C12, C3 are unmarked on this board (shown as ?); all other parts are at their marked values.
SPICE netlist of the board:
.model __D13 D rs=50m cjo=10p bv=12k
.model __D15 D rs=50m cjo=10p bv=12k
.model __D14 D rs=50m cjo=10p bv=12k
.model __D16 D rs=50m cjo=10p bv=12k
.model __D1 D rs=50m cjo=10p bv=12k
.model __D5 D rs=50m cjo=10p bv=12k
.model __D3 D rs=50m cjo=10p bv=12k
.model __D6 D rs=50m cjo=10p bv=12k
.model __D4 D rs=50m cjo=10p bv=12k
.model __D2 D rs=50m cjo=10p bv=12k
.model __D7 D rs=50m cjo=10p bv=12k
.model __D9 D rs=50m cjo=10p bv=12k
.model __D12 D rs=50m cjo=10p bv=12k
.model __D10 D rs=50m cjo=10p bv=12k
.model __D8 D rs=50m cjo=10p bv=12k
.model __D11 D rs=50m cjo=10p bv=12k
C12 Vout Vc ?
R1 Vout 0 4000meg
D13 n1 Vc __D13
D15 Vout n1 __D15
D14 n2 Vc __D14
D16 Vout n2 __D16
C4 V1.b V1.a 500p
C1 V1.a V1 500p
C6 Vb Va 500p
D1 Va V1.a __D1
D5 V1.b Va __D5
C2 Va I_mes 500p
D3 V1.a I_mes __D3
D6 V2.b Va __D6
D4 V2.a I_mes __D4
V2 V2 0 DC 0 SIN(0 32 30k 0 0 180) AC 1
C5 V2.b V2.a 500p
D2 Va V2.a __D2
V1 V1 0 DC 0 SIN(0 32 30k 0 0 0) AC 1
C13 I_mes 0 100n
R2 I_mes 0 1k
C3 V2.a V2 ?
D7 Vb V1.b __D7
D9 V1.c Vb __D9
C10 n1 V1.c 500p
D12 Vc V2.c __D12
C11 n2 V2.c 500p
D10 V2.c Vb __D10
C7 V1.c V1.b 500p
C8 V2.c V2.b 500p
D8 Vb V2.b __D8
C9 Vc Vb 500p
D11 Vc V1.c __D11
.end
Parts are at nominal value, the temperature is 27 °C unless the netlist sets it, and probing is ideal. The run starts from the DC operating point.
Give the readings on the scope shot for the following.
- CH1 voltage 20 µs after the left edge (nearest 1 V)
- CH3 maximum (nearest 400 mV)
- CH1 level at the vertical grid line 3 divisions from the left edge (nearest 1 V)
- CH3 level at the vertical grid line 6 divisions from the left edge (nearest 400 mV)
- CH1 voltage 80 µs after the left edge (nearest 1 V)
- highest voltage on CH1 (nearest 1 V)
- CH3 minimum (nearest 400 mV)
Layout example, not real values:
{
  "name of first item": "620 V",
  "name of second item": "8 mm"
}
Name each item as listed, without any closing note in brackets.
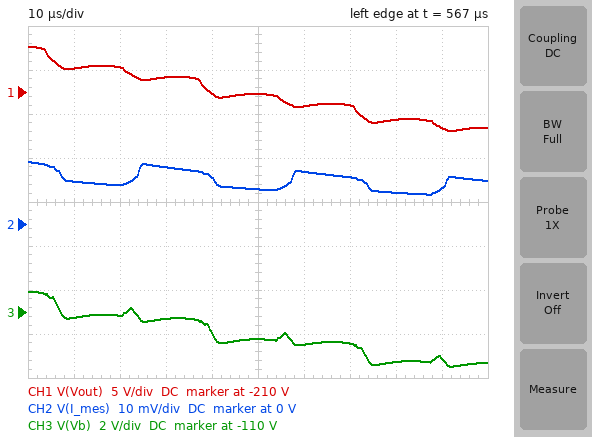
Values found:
{
  "CH1 voltage 20 µs after the left edge": "-207 V",
  "CH3 maximum": "-109.2 V",
  "CH1 level at the vertical grid line 3 divisions from the left edge": "-208 V",
  "CH3 level at the vertical grid line 6 divisions from the left edge": "-111.6 V",
  "CH1 voltage 80 µs after the left edge": "-213 V",
  "highest voltage on CH1": "-205 V",
  "CH3 minimum": "-112.4 V"
}
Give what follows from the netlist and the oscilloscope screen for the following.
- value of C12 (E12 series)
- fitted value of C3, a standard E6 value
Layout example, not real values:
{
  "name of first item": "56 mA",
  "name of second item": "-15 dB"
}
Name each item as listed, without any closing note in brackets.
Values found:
{
  "value of C12": "270 pF",
  "fitted value of C3, a standard E6 value": "680 pF"
}
